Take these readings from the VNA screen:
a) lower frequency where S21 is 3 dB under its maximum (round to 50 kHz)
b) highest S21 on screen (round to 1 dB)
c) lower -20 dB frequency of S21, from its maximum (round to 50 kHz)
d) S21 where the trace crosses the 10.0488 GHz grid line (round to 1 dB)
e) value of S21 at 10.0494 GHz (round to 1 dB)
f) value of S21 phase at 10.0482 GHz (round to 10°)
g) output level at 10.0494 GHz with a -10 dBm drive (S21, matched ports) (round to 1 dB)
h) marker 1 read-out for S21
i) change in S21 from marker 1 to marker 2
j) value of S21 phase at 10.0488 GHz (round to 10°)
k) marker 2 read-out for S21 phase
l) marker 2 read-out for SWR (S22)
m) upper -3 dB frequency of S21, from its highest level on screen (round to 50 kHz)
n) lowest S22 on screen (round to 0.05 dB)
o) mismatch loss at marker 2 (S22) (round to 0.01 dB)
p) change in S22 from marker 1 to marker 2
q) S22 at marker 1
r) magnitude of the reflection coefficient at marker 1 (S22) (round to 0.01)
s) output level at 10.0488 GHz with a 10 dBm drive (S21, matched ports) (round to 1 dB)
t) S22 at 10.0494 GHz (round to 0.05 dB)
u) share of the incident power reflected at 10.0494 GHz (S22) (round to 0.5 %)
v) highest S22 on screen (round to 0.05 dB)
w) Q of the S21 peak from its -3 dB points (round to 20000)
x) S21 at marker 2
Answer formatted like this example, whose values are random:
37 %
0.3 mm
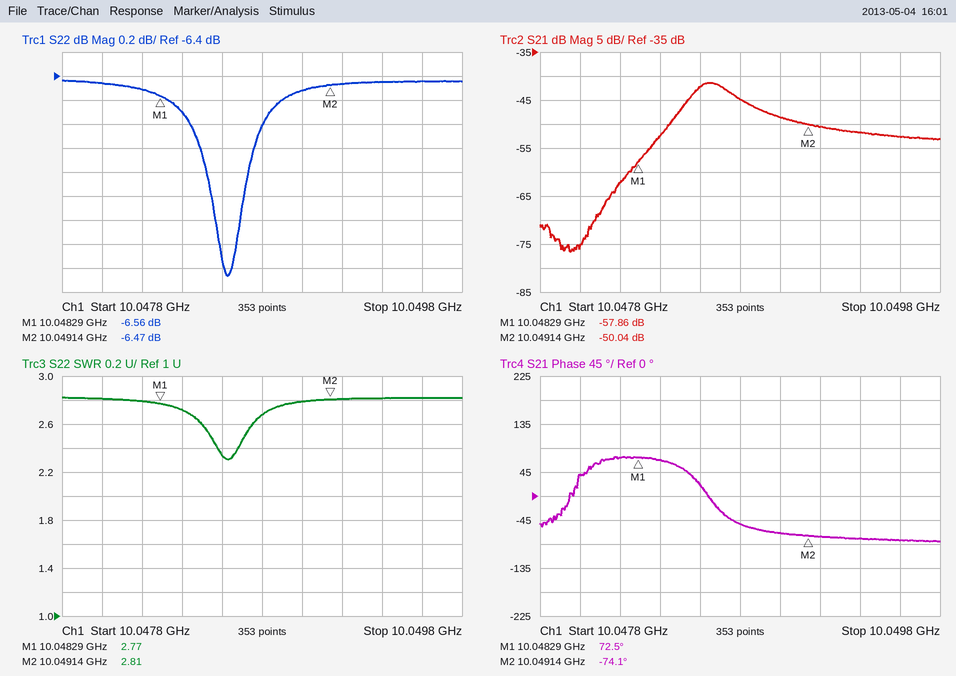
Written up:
10.04855 GHz
-41 dB
10.04820 GHz
-45 dB
-52 dB
70°
-62 dBm
-57.86 dB
7.82 dB
-50°
-74.1°
2.81
10.04880 GHz
-8.05 dB
1.11 dB
0.09 dB
-6.56 dB
0.47
-35 dBm
-6.45 dB
22.5 %
-6.45 dB
40000
-50.04 dB
